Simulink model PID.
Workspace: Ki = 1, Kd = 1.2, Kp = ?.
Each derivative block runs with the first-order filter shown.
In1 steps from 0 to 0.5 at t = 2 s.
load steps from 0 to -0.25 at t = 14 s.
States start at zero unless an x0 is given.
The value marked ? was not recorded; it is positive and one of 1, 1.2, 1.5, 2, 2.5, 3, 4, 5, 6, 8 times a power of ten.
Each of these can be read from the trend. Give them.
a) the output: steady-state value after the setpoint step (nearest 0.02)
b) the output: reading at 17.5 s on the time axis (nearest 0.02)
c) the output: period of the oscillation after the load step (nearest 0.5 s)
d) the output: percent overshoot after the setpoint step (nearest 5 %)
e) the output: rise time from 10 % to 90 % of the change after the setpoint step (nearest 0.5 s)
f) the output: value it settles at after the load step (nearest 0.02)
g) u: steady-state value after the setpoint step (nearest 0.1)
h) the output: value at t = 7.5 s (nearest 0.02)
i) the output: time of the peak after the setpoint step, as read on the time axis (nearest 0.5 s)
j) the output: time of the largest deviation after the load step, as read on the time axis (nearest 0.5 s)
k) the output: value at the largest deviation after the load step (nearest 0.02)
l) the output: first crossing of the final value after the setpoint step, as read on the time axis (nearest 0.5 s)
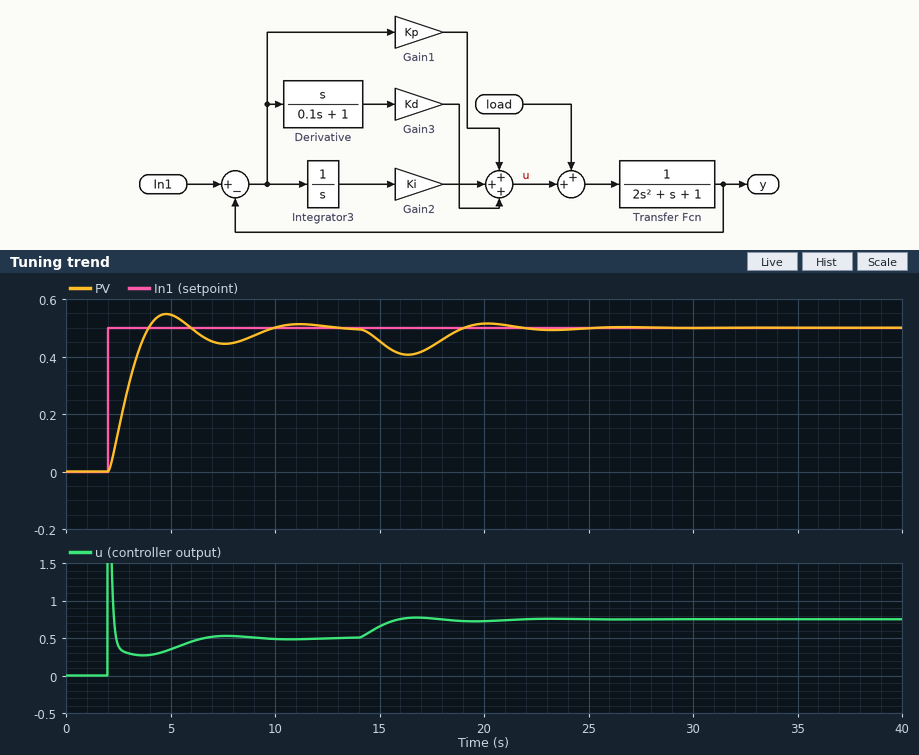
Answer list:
0.50
0.44
7.0 s
10 %
1.5 s
0.50
0.5
0.44
5.0 s
16.5 s
0.40
4.0 s
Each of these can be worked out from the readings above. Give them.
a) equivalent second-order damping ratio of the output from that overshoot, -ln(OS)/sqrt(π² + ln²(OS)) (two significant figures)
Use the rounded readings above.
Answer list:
0.59
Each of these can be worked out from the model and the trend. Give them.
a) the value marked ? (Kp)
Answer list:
1.5
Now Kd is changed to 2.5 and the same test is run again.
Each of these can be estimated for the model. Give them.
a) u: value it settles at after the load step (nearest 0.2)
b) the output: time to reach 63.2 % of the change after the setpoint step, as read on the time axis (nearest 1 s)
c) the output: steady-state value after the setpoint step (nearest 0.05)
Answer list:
0.8
3 s
0.50
